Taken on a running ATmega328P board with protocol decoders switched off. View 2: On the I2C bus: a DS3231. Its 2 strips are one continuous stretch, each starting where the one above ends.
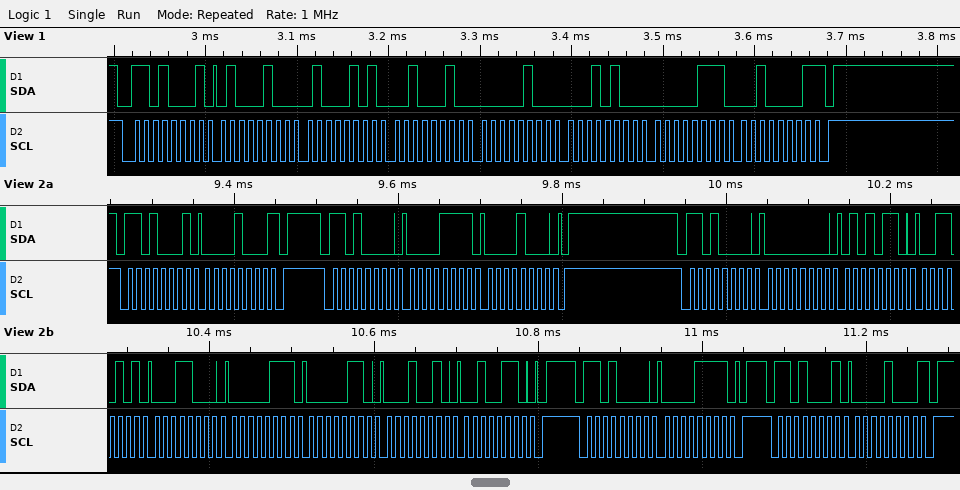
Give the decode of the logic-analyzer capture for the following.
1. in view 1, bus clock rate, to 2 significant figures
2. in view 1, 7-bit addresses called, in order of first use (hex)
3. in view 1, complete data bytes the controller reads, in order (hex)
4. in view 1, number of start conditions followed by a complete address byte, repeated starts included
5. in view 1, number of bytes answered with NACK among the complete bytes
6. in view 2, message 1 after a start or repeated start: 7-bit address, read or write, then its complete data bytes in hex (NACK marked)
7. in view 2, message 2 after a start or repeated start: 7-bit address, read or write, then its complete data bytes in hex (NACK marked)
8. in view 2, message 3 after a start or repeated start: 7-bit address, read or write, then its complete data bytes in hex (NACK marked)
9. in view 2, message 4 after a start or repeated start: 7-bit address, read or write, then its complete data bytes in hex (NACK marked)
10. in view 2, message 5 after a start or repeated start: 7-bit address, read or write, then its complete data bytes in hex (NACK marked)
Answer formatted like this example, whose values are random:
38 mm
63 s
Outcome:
100 kHz
0x68
44 45 22 04 14 07 21
1
1
0x68 read: 08 NACK
0x68 write: 0F 08
0x68 write: 00 56 35 18 07 06 12 26
0x68 write: 0F
0x68 read: 08 NACK
